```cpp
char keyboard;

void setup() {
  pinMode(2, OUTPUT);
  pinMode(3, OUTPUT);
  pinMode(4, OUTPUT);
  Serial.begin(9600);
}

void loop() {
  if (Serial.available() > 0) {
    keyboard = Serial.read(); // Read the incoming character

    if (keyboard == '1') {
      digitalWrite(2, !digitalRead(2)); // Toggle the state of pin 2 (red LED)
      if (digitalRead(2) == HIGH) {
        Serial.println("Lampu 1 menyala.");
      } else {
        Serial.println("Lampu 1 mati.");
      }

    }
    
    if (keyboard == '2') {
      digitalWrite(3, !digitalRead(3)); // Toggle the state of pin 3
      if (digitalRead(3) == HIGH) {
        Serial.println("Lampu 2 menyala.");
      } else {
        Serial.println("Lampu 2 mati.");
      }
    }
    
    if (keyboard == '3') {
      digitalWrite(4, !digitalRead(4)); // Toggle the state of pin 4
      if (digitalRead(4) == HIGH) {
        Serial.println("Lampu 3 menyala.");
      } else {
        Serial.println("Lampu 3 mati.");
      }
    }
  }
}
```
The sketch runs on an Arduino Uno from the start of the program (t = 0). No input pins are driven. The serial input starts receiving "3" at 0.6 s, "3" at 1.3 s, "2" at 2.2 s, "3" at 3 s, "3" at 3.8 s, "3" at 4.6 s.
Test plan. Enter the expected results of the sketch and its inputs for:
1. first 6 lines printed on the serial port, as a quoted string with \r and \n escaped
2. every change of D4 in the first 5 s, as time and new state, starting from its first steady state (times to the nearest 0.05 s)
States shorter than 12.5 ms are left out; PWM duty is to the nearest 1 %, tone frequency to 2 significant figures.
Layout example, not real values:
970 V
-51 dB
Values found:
"Lampu 3 menyala.\r\nLampu 3 mati.\r\nLampu 2 menyala.\r\nLampu 3 menyala.\r\nLampu 3 mati.\r\nLampu 3 menyala.\r\n"
0 s low; 0.6 s high; 1.3 s low; 3 s high; 3.8 s low; 4.6 s high
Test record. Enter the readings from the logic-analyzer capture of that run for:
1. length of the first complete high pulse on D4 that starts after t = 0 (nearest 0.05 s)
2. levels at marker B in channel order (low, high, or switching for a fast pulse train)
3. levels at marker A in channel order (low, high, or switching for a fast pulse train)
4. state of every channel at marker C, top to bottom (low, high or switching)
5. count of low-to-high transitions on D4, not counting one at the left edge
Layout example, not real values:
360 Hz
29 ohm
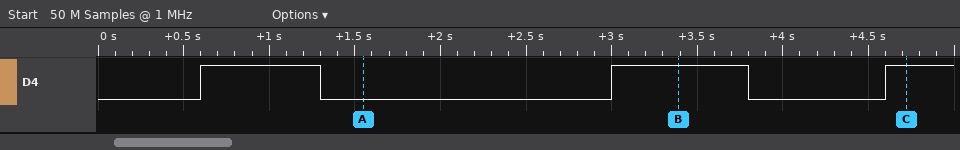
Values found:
0.70 s
D4 high
D4 low
D4 high
3
